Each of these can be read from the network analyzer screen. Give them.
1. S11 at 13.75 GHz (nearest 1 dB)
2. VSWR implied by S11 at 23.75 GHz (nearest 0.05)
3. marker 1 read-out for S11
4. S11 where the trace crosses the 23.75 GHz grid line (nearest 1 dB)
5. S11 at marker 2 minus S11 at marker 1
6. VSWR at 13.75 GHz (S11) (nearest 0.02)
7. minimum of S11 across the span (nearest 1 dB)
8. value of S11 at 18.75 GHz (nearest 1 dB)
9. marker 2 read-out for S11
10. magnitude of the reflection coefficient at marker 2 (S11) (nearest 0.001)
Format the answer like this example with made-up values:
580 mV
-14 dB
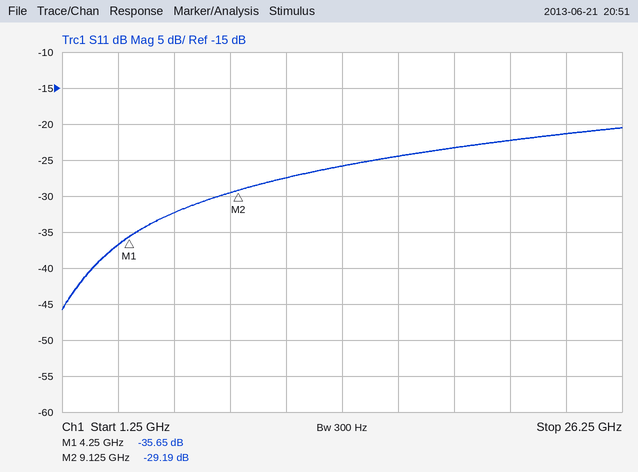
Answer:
-26 dB
1.20
-35.65 dB
-21 dB
6.46 dB
1.10
-46 dB
-23 dB
-29.19 dB
0.035
